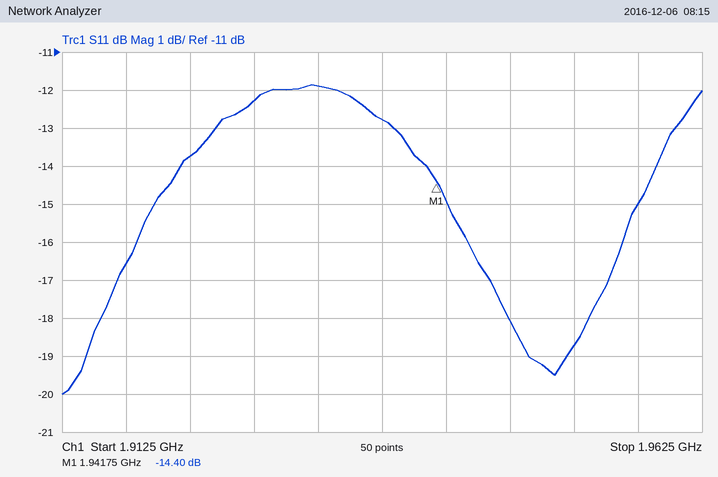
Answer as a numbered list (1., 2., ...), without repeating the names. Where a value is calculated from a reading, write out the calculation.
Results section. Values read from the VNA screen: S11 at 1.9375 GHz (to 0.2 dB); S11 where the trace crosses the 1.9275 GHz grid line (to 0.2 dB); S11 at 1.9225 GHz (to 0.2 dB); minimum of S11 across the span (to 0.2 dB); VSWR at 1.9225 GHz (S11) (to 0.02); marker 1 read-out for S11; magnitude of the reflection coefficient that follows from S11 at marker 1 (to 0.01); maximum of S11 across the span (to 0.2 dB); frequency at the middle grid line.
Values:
1. -12.8 dB
2. -12.2 dB
3. -13.8 dB
4. -20.0 dB
5. |Γ| = 10^(-13.8/20) = 0.2042; VSWR = (1 + 0.2042)/(1 − 0.2042) ≈ 1.51, so 1.52 to the nearest 0.02
6. -14.40 dB
7. 10^(-14.4/20) ≈ 0.19
8. -11.8 dB
9. 1.9375 GHz
